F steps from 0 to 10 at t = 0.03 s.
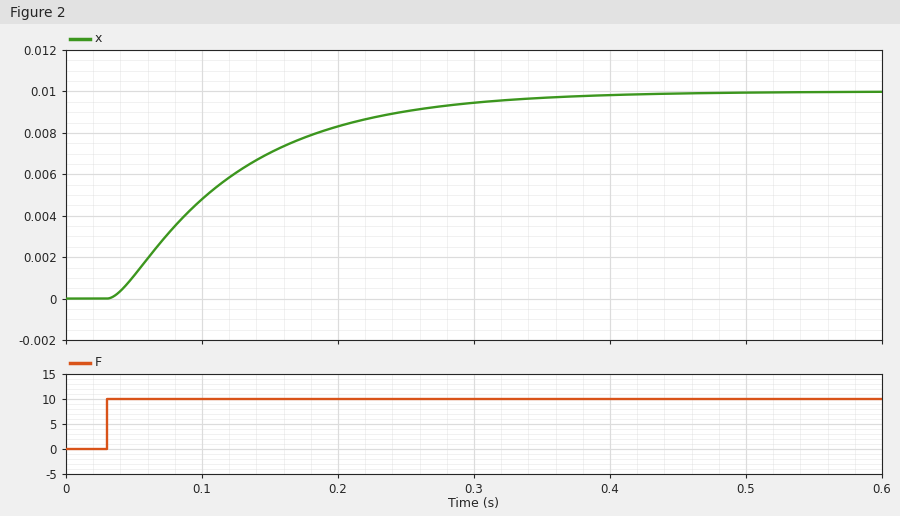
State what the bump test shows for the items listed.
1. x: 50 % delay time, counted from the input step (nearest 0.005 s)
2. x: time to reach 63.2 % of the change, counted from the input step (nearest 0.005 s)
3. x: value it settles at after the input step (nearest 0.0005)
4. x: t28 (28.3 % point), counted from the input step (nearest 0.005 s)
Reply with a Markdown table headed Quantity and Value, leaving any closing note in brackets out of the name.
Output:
| Quantity | Value |
|---|---|
| x: 50 % delay time, counted from the input step | 0.075 s |
| x: time to reach 63.2 % of the change, counted from the input step | 0.100 s |
| x: value it settles at after the input step | 0.0100 |
| x: t28 (28.3 % point), counted from the input step | 0.040 s |
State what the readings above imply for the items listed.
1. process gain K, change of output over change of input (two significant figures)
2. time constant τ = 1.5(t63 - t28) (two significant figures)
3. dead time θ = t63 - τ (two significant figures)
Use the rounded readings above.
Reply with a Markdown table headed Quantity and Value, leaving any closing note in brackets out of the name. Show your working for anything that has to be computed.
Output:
| Quantity | Value |
|---|---|
| process gain K, change of output over change of input | (0.01 - 0) / 10 = 0.0010 |
| time constant τ = 1.5(t63 - t28) | 1.5 × (0.1 - 0.04) = 0.090 s |
| dead time θ = t63 - τ | 0.1 - 0.09 = 0.010 s |
